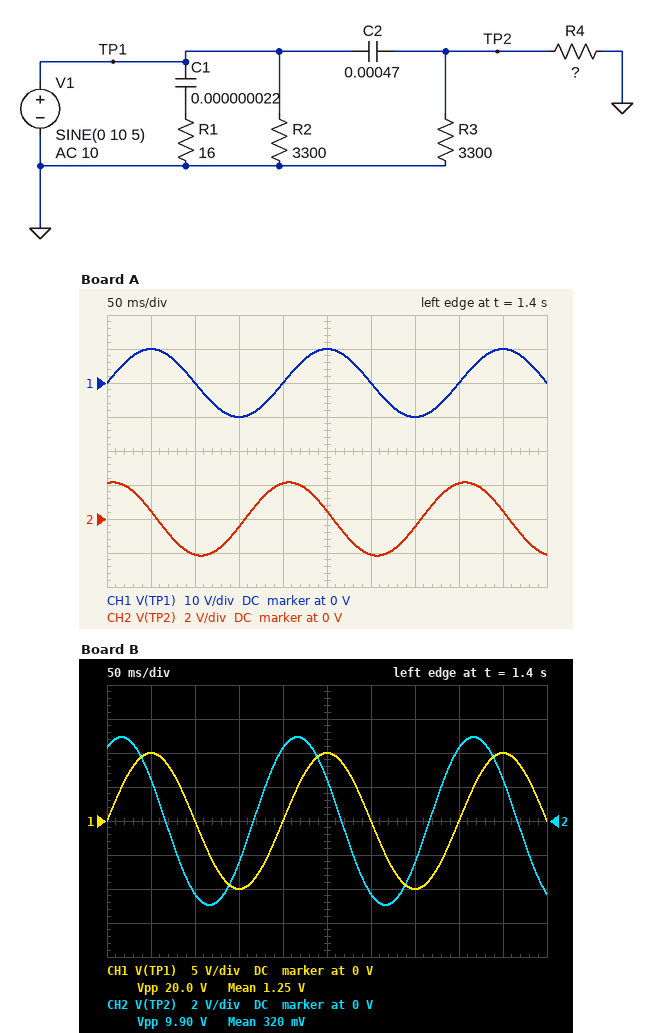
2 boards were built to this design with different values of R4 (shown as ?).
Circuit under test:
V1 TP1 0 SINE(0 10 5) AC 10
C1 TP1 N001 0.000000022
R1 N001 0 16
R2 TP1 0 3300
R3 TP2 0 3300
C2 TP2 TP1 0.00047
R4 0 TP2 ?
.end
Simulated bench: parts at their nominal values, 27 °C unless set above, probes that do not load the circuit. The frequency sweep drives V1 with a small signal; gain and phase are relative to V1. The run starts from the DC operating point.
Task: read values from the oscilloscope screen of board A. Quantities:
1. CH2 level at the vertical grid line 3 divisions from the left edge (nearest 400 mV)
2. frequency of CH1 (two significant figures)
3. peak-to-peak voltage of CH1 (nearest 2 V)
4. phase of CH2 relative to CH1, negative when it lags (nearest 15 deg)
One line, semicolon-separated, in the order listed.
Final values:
-400 mV; 5.0 Hz; 20 V; 75 deg
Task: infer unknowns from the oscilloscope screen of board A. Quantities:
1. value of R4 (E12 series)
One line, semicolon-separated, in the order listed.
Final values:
15 Ω
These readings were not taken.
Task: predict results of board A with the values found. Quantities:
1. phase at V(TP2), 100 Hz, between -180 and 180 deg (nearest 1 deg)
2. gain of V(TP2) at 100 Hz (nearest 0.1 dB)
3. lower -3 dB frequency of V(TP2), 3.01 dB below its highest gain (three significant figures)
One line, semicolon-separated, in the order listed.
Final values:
13 deg; -0.2 dB; 22.7 Hz
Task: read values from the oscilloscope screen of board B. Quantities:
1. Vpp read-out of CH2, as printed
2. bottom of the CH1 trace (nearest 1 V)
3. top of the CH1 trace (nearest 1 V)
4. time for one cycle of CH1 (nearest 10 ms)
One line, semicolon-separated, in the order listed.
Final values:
9.90 V; -10 V; 10 V; 200 ms
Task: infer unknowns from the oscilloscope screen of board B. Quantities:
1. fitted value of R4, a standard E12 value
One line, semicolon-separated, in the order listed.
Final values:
39 Ω
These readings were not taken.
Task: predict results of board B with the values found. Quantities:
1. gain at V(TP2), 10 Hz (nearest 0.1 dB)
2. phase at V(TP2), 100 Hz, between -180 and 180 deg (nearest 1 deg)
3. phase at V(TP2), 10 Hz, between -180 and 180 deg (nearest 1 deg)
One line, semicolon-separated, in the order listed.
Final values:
-2.5 dB; 5 deg; 41 deg
